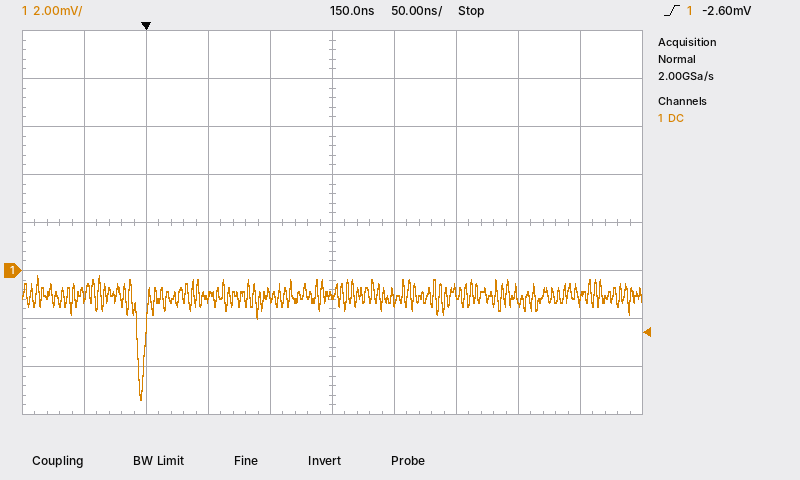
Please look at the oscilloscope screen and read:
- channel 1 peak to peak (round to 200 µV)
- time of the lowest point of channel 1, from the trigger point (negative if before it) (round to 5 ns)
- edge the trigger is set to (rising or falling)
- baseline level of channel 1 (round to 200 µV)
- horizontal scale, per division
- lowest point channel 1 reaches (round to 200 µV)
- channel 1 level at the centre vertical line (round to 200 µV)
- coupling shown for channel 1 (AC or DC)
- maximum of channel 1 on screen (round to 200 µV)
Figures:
5.2 mV
-5 ns
rising
-1.0 mV
50 ns
-5.4 mV
-1.0 mV
DC
-200 µV
